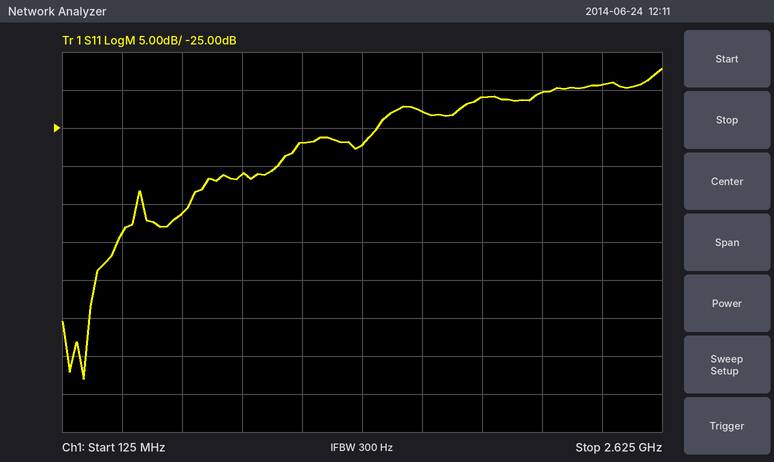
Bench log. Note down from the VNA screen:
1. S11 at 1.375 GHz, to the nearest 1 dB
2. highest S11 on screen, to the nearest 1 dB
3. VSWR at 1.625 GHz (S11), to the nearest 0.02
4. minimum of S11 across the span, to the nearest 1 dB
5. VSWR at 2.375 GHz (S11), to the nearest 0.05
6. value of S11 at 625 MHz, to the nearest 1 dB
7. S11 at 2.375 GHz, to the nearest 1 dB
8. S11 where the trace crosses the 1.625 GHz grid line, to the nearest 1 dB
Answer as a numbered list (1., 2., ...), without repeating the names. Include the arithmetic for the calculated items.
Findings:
1. -27 dB
2. -17 dB
3. |Γ| = 10^(-23/20) = 0.0708; VSWR = (1 + 0.0708)/(1 − 0.0708) ≈ 1.15, so 1.16 to the nearest 0.02
4. -58 dB
5. |Γ| = 10^(-19/20) = 0.1122; VSWR = (1 + 0.1122)/(1 − 0.1122) ≈ 1.25
6. -36 dB
7. -19 dB
8. -23 dB
